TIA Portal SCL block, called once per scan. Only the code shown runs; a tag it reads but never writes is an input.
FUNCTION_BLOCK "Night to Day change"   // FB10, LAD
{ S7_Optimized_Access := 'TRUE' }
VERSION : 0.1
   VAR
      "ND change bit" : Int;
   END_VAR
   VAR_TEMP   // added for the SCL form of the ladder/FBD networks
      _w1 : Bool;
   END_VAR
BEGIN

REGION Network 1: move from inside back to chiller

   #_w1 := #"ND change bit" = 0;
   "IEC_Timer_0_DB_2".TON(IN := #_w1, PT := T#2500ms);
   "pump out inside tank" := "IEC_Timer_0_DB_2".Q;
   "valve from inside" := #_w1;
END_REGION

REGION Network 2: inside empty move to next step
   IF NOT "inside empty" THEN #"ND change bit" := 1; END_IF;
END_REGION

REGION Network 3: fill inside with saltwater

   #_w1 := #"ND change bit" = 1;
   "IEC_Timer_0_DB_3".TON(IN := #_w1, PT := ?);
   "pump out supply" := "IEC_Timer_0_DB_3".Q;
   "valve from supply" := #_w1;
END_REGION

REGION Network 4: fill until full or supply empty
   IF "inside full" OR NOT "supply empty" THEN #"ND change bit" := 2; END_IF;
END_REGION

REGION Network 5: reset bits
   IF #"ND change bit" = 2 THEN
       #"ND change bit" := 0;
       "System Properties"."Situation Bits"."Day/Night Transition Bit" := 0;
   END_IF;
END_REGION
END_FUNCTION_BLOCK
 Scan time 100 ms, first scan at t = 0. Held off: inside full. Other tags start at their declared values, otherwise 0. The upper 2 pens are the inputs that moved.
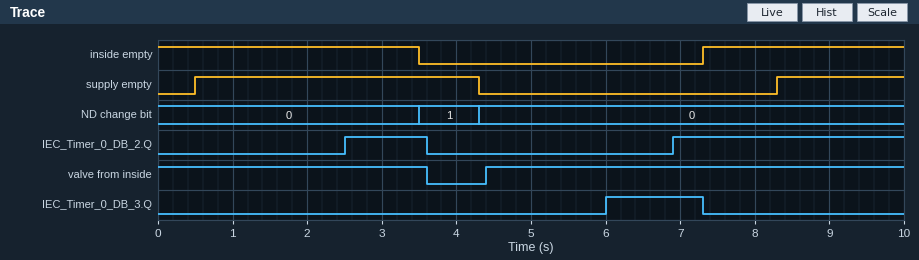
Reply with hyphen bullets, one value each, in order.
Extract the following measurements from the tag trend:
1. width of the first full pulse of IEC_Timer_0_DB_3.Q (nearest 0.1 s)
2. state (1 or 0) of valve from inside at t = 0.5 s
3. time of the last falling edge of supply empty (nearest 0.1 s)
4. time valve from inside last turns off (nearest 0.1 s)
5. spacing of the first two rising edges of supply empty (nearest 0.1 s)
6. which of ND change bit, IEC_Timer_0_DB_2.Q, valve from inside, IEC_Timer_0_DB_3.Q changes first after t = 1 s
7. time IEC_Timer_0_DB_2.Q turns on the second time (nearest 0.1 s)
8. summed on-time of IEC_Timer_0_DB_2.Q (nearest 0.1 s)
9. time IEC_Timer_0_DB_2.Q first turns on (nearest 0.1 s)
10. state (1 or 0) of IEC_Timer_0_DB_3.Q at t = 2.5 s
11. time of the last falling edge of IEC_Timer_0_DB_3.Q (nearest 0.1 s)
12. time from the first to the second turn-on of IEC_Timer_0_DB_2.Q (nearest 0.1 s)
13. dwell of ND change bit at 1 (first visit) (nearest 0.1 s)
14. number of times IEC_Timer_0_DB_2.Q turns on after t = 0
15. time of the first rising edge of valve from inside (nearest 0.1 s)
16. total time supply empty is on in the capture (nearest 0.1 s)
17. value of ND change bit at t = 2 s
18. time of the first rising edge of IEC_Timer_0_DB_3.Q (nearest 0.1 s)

- 1.3 s
- 1
- 4.3 s
- 3.6 s
- 7.8 s
- IEC_Timer_0_DB_2.Q
- 6.9 s
- 4.2 s
- 2.5 s
- 0
- 7.3 s
- 4.4 s
- 0.8 s
- 2
- 4.4 s
- 5.5 s
- 0
- 6.0 s
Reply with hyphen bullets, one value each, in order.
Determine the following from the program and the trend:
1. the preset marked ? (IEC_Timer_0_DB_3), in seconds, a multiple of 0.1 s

- 2.5 s
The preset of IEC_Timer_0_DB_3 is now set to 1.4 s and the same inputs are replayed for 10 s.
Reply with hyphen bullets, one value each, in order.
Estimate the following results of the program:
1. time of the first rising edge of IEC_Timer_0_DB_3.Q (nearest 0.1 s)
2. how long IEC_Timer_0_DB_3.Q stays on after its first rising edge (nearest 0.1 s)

- 4.9 s
- 2.4 s
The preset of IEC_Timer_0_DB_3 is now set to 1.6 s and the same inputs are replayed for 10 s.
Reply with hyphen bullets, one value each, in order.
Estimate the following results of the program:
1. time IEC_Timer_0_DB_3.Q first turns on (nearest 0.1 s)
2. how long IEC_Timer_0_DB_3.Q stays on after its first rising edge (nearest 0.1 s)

- 5.1 s
- 2.2 s
